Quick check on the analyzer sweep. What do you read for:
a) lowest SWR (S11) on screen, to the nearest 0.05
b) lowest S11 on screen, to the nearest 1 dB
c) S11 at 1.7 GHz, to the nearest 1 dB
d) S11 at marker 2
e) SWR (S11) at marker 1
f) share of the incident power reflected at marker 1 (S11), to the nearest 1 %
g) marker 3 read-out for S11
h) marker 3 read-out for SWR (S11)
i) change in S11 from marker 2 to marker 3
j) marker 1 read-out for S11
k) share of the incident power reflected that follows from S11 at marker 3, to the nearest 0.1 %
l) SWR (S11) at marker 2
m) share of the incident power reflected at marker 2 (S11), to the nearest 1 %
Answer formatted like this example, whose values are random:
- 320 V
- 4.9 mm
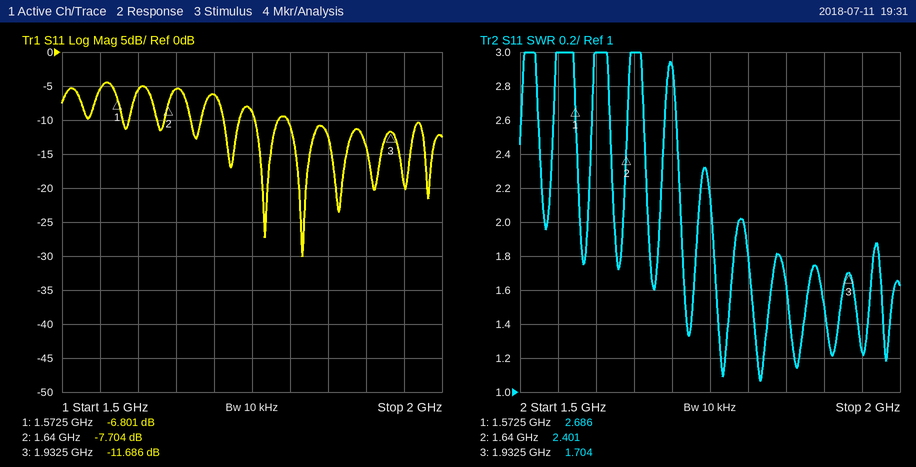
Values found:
- 1.05
- -30 dB
- -6 dB
- -7.704 dB
- 2.686
- 21 %
- -11.686 dB
- 1.704
- -3.982 dB
- -6.801 dB
- 6.8 %
- 2.401
- 17 %
